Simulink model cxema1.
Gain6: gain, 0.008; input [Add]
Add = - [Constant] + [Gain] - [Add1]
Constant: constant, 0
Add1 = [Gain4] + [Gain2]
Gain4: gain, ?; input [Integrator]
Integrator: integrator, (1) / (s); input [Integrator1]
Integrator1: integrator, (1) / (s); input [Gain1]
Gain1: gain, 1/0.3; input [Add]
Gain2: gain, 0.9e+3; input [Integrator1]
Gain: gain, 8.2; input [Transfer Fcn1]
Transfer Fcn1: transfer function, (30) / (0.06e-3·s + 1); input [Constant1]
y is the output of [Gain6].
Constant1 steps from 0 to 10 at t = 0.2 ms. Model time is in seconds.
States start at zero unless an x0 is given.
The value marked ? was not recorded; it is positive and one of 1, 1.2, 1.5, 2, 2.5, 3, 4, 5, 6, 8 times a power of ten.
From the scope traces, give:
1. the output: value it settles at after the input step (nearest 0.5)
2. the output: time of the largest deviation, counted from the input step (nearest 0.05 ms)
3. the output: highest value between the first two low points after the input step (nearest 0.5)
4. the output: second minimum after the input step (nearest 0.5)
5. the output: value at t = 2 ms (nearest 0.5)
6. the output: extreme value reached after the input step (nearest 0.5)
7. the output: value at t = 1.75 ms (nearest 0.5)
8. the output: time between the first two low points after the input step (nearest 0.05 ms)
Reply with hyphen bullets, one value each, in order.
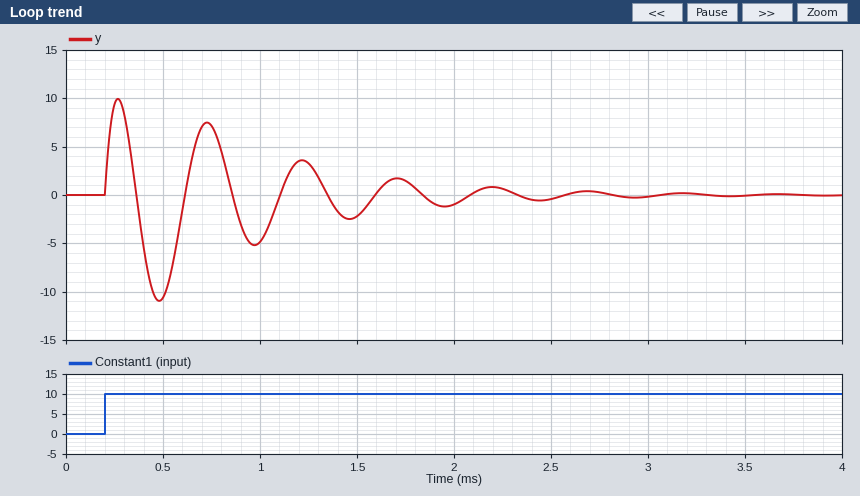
- 0.0
- 0.30 ms
- 7.5
- -5.0
- -1.0
- -11.0
- 1.5
- 0.50 ms
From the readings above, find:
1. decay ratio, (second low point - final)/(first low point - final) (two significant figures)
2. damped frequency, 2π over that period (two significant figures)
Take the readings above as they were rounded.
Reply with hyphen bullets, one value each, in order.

- 0.45
- 13 rad/ms
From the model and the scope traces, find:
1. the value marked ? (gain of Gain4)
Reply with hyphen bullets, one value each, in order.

- 5e+07
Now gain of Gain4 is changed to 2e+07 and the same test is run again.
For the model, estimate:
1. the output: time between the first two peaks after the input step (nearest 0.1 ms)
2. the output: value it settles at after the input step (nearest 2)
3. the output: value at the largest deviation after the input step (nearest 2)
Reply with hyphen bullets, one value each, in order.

- 0.7 ms
- 0
- 12
